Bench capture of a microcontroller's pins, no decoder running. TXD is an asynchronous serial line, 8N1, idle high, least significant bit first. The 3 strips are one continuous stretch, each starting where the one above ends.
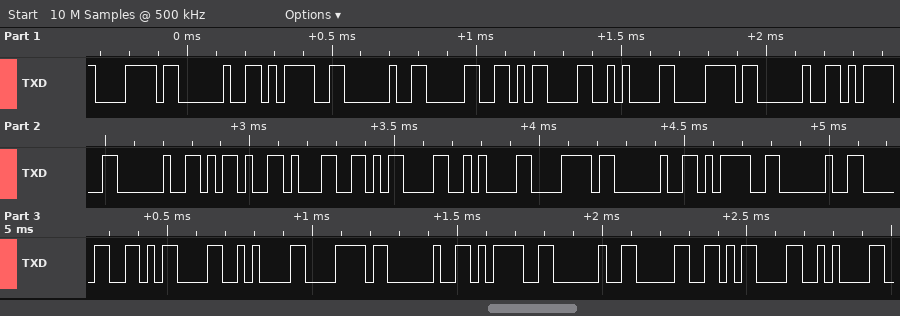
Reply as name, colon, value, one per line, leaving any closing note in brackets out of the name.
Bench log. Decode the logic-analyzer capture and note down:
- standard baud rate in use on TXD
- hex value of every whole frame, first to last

standard baud rate in use on TXD: 38400 baud
hex value of every whole frame, first to last: 78 20 3D 20 30 0D 0A 78 20 3D 20 2D 31 0D 0A 78 20 3D 20 30 0D 0A 78 20 3D 20 30 0D 0A
